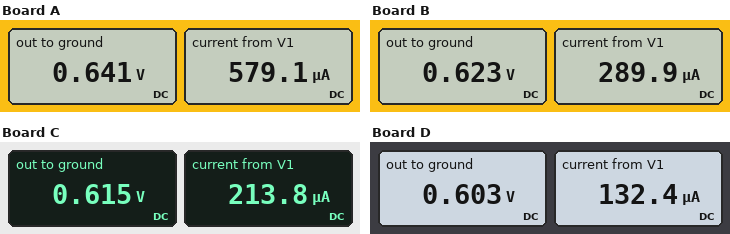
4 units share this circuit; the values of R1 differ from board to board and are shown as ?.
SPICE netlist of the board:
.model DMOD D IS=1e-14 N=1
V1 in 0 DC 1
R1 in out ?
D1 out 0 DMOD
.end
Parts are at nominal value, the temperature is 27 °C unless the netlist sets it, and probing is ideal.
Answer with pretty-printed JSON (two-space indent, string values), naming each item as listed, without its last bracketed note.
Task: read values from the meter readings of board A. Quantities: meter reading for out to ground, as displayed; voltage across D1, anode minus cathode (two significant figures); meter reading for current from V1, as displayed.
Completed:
{
  "meter reading for out to ground, as displayed": "0.641 V",
  "voltage across D1, anode minus cathode": "640 mV",
  "meter reading for current from V1, as displayed": "579.1 µA"
}
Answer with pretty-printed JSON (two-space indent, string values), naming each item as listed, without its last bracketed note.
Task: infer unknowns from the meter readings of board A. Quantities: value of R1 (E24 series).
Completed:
{
  "value of R1": "620 Ω"
}
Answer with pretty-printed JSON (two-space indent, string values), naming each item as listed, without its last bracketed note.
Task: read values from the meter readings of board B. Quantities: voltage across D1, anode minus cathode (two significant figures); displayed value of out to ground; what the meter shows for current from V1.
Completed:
{
  "voltage across D1, anode minus cathode": "620 mV",
  "displayed value of out to ground": "0.623 V",
  "what the meter shows for current from V1": "289.9 µA"
}
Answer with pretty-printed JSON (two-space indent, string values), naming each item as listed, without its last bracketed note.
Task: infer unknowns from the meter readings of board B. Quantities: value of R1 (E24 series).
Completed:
{
  "value of R1": "1.3 kΩ"
}
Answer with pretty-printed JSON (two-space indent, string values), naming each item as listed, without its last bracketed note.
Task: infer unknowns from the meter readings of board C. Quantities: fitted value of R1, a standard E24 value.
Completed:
{
  "fitted value of R1, a standard E24 value": "1.8 kΩ"
}
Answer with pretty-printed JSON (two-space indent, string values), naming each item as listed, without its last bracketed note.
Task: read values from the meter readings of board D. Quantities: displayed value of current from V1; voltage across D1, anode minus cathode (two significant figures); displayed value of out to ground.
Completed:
{
  "displayed value of current from V1": "132.4 µA",
  "voltage across D1, anode minus cathode": "600 mV",
  "displayed value of out to ground": "0.603 V"
}
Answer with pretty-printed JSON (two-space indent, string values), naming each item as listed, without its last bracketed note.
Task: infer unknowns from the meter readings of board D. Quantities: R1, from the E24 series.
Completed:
{
  "R1, from the E24 series": "3 kΩ"
}
